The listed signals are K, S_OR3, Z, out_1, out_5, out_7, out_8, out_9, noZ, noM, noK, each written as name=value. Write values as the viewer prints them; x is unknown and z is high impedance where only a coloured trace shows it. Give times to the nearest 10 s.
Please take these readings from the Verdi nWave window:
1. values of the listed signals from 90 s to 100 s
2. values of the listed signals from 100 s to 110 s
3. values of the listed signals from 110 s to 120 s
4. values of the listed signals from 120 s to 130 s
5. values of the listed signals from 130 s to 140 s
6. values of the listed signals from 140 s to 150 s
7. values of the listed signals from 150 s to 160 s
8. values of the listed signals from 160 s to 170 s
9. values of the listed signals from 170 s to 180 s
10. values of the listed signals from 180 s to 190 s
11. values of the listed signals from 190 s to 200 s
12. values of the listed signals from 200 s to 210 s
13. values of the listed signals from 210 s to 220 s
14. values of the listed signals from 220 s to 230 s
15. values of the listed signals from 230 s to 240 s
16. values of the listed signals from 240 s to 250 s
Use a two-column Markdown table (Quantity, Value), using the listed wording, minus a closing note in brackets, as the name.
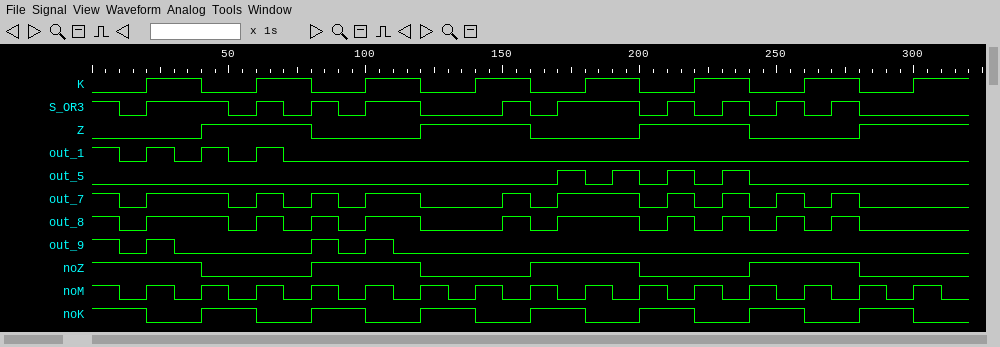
| Quantity | Value |
|---|---|
| values of the listed signals from 90 s to 100 s | K=0, S_OR3=0, Z=0, out_1=0, out_5=0, out_7=0, out_8=0, out_9=0, noZ=1, noM=0, noK=1 |
| values of the listed signals from 100 s to 110 s | K=1, S_OR3=1, Z=0, out_1=0, out_5=0, out_7=1, out_8=1, out_9=1, noZ=1, noM=1, noK=0 |
| values of the listed signals from 110 s to 120 s | K=1, S_OR3=1, Z=0, out_1=0, out_5=0, out_7=1, out_8=1, out_9=0, noZ=1, noM=0, noK=0 |
| values of the listed signals from 120 s to 130 s | K=0, S_OR3=0, Z=1, out_1=0, out_5=0, out_7=0, out_8=0, out_9=0, noZ=0, noM=1, noK=1 |
| values of the listed signals from 130 s to 140 s | K=0, S_OR3=0, Z=1, out_1=0, out_5=0, out_7=0, out_8=0, out_9=0, noZ=0, noM=0, noK=1 |
| values of the listed signals from 140 s to 150 s | K=1, S_OR3=0, Z=1, out_1=0, out_5=0, out_7=0, out_8=0, out_9=0, noZ=0, noM=1, noK=0 |
| values of the listed signals from 150 s to 160 s | K=1, S_OR3=1, Z=1, out_1=0, out_5=0, out_7=1, out_8=1, out_9=0, noZ=0, noM=0, noK=0 |
| values of the listed signals from 160 s to 170 s | K=0, S_OR3=0, Z=0, out_1=0, out_5=0, out_7=0, out_8=0, out_9=0, noZ=1, noM=1, noK=1 |
| values of the listed signals from 170 s to 180 s | K=0, S_OR3=1, Z=0, out_1=0, out_5=1, out_7=1, out_8=1, out_9=0, noZ=1, noM=0, noK=1 |
| values of the listed signals from 180 s to 190 s | K=1, S_OR3=1, Z=0, out_1=0, out_5=0, out_7=1, out_8=1, out_9=0, noZ=1, noM=1, noK=0 |
| values of the listed signals from 190 s to 200 s | K=1, S_OR3=1, Z=0, out_1=0, out_5=1, out_7=1, out_8=1, out_9=0, noZ=1, noM=0, noK=0 |
| values of the listed signals from 200 s to 210 s | K=0, S_OR3=0, Z=1, out_1=0, out_5=0, out_7=0, out_8=0, out_9=0, noZ=0, noM=1, noK=1 |
| values of the listed signals from 210 s to 220 s | K=0, S_OR3=1, Z=1, out_1=0, out_5=1, out_7=1, out_8=1, out_9=0, noZ=0, noM=0, noK=1 |
| values of the listed signals from 220 s to 230 s | K=1, S_OR3=0, Z=1, out_1=0, out_5=0, out_7=0, out_8=0, out_9=0, noZ=0, noM=1, noK=0 |
| values of the listed signals from 230 s to 240 s | K=1, S_OR3=1, Z=1, out_1=0, out_5=1, out_7=1, out_8=1, out_9=0, noZ=0, noM=0, noK=0 |
| values of the listed signals from 240 s to 250 s | K=0, S_OR3=0, Z=0, out_1=0, out_5=0, out_7=0, out_8=0, out_9=0, noZ=1, noM=1, noK=1 |
